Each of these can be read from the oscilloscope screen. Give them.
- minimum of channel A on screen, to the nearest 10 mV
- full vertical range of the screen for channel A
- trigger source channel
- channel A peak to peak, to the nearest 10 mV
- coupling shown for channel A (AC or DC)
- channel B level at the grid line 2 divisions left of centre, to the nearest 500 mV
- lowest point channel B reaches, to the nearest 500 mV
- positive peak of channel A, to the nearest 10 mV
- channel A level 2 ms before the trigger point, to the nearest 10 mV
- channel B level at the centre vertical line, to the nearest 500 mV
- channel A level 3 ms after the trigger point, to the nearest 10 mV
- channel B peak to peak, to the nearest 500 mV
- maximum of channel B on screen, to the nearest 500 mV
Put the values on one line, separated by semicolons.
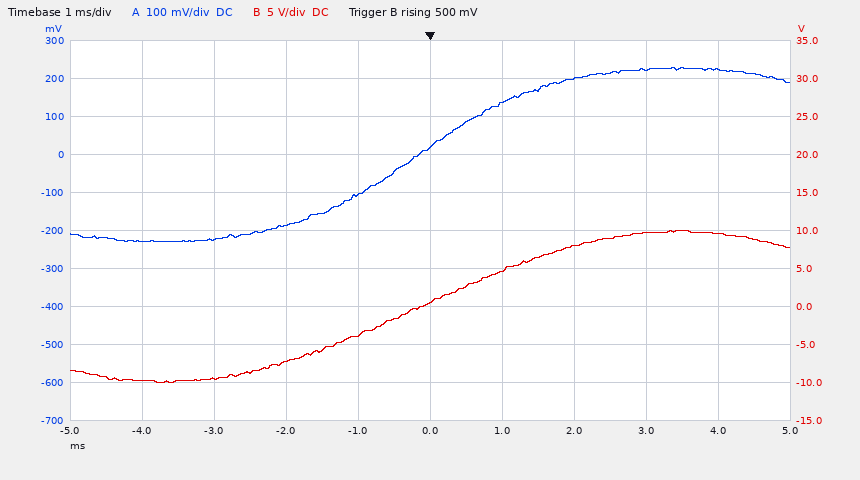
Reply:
-230 mV; 1 V; channel B; 460 mV; DC; -7.0 V; -10.0 V; 230 mV; -190 mV; 500 mV; 220 mV; 20.0 V; 10.0 V
